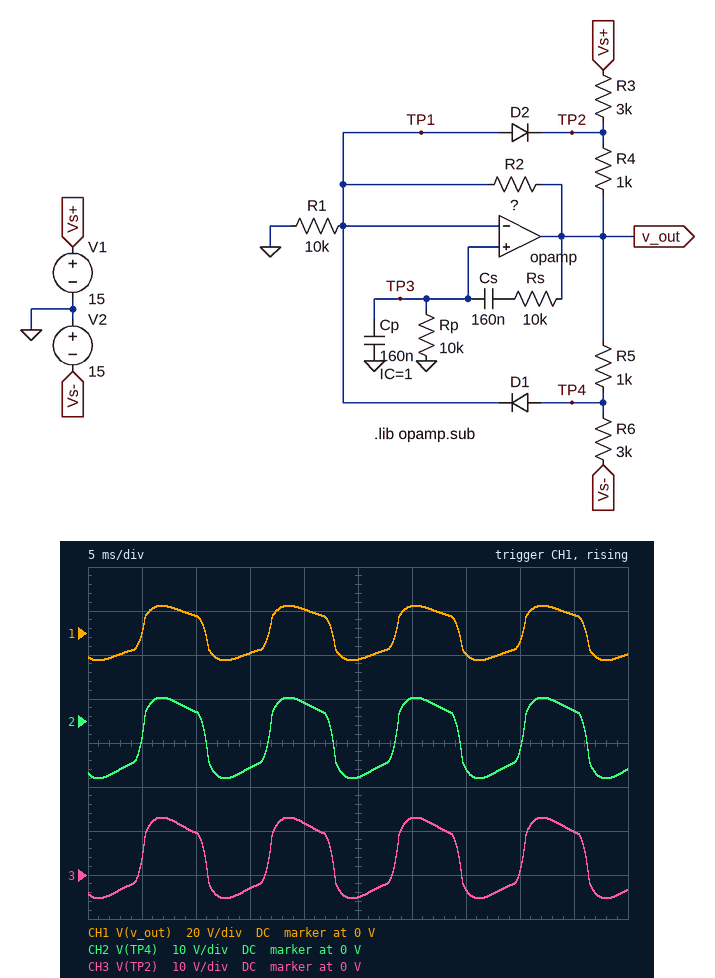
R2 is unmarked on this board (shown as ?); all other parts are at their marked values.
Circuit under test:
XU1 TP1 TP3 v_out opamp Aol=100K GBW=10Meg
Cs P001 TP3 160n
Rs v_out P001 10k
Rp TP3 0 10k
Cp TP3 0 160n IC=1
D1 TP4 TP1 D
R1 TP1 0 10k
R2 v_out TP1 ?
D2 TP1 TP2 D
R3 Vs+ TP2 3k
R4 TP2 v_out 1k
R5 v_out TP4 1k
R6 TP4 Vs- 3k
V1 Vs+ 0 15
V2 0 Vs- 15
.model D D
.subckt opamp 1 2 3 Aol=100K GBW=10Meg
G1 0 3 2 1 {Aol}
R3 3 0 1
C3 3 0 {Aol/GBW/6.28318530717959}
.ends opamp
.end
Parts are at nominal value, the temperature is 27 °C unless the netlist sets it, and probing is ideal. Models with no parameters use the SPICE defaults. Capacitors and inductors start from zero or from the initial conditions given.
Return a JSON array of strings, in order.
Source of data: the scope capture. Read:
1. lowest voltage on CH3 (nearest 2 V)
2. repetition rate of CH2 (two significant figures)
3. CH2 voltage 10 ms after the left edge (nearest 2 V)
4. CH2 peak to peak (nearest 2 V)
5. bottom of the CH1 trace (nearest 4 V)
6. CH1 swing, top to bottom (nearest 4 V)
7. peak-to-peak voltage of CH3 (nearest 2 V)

["-6 V", "85 Hz", "2 V", "18 V", "-12 V", "24 V", "18 V"]
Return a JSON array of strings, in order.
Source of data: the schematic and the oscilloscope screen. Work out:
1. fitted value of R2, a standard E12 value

["47 kΩ"]
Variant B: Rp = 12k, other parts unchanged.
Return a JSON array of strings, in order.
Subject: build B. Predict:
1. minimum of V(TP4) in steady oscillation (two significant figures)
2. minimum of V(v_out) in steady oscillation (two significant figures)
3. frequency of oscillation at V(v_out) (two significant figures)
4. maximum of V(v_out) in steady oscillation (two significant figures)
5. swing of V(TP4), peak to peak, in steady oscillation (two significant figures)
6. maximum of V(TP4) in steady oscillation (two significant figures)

["-14 V", "-13 V", "77 Hz", "13 V", "20 V", "5.9 V"]
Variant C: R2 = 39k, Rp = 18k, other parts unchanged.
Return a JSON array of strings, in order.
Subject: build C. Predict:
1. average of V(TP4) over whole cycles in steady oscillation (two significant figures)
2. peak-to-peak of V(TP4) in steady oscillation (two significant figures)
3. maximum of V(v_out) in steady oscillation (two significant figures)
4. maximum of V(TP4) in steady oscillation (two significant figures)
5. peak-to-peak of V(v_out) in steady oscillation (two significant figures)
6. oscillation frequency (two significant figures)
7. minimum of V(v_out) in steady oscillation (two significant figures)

["-3.8 V", "22 V", "15 V", "7.2 V", "30 V", "63 Hz", "-15 V"]
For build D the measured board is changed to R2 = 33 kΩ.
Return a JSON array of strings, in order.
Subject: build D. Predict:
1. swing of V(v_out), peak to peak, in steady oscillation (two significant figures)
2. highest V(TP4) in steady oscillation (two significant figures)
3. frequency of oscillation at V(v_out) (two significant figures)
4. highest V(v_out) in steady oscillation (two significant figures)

["24 V", "5.1 V", "91 Hz", "12 V"]
